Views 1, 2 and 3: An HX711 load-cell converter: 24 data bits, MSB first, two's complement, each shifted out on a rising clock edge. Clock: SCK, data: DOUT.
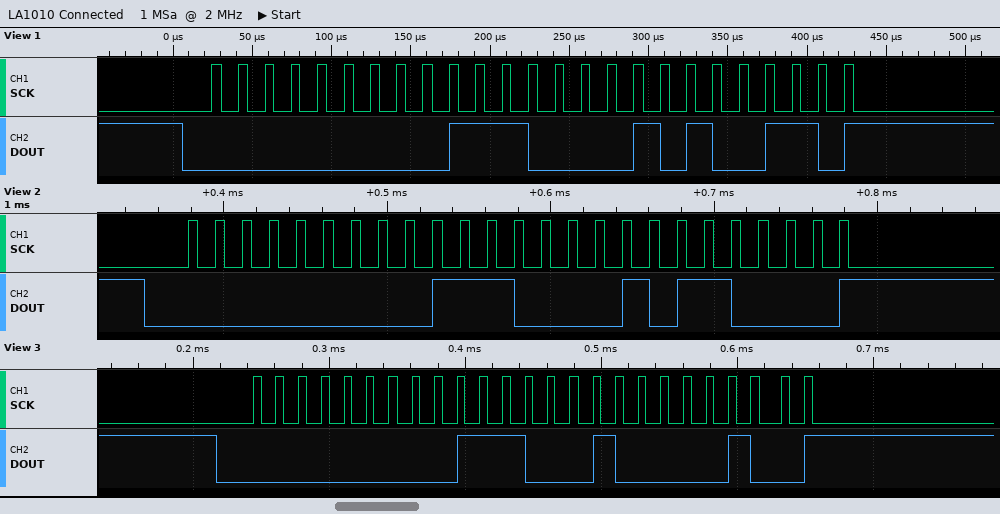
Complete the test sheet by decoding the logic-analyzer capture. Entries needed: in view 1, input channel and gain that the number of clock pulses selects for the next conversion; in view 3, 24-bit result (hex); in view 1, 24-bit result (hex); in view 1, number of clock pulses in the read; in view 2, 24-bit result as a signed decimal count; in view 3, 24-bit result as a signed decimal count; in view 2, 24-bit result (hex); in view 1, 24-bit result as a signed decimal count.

channel A, gain 128
0x007104
0x0070A6
25
28848
28932
0x0070B0
28838
